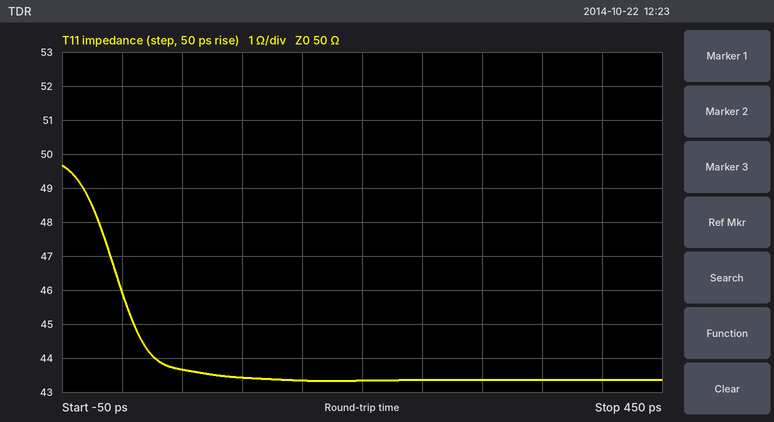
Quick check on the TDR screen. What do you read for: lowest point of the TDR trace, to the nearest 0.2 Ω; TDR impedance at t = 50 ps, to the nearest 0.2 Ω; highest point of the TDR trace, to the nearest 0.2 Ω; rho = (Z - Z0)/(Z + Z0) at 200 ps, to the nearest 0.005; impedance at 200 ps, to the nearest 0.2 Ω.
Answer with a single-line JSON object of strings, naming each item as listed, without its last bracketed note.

{"lowest point of the TDR trace, to the nearest 0.2 Ω": "43.4 Ω", "TDR impedance at t = 50 ps, to the nearest 0.2 Ω": "43.6 Ω", "highest point of the TDR trace, to the nearest 0.2 Ω": "49.6 Ω", "rho = (Z - Z0)/(Z + Z0) at 200 ps, to the nearest 0.005": "-0.070", "impedance at 200 ps, to the nearest 0.2 Ω": "43.4 Ω"}
